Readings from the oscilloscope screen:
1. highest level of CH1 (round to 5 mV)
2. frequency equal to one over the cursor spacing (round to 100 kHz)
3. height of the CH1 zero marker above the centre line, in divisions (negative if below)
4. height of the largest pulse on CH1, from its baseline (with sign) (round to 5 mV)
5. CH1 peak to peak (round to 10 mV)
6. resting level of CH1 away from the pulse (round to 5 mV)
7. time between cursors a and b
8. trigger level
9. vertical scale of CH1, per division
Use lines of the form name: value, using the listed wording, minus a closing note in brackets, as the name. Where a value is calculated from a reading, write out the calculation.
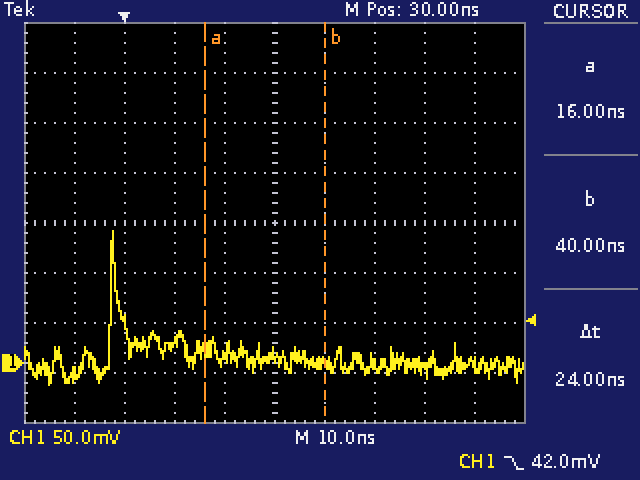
highest level of CH1: 130 mV
frequency equal to one over the cursor spacing: 1 / 24 ns ≈ 41.7 MHz
height of the CH1 zero marker above the centre line, in divisions: -2.8 div
height of the largest pulse on CH1, from its baseline (with sign): 130 mV − (0 mV) = +130 mV
CH1 peak to peak: 150 mV
resting level of CH1 away from the pulse: 0 mV
time between cursors a and b: 24 ns
trigger level: 42.0 mV
vertical scale of CH1, per division: 50 mV
